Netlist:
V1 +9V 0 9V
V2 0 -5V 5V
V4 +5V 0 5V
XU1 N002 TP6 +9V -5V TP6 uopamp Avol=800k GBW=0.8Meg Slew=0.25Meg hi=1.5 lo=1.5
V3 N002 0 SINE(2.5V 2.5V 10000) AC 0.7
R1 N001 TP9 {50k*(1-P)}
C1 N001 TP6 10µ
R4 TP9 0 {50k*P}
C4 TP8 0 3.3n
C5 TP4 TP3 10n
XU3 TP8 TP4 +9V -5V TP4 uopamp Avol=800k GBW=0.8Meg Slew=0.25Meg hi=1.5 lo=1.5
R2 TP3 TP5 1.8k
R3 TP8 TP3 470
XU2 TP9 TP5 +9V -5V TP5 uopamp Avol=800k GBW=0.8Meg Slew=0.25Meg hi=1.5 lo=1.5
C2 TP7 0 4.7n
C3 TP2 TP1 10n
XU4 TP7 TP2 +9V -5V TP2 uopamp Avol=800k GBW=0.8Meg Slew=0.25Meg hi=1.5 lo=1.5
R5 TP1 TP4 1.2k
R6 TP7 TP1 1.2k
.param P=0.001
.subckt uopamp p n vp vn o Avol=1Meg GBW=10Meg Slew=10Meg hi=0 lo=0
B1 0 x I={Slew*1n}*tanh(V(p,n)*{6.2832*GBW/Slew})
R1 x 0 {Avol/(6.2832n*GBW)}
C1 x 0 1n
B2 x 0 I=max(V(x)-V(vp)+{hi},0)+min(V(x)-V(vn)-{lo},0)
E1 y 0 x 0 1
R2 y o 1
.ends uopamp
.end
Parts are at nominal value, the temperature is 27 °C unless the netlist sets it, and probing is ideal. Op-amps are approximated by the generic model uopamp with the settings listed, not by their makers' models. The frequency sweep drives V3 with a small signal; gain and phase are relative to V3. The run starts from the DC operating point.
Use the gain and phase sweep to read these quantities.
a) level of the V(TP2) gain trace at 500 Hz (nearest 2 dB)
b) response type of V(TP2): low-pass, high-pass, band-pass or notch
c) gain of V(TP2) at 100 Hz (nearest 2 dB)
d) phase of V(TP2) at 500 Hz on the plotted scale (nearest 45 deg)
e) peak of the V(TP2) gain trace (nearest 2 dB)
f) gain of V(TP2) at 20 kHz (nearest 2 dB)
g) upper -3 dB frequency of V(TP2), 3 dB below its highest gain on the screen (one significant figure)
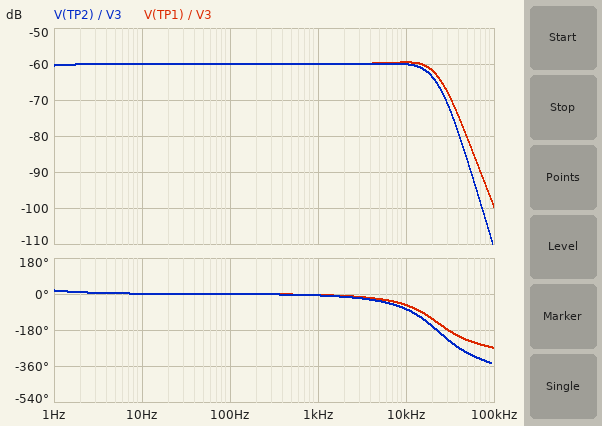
-60 dB
low-pass
-60 dB
0 deg
-60 dB
-64 dB
20 kHz
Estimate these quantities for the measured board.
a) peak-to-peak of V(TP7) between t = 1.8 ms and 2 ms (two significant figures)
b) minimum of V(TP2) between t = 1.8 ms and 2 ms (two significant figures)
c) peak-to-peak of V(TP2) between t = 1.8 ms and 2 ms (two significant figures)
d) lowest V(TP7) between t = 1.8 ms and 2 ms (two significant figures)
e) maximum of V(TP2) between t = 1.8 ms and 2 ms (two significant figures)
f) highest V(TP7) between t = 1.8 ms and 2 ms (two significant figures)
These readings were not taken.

5.0 mV
-2.5 mV
5.0 mV
-2.5 mV
2.5 mV
2.5 mV
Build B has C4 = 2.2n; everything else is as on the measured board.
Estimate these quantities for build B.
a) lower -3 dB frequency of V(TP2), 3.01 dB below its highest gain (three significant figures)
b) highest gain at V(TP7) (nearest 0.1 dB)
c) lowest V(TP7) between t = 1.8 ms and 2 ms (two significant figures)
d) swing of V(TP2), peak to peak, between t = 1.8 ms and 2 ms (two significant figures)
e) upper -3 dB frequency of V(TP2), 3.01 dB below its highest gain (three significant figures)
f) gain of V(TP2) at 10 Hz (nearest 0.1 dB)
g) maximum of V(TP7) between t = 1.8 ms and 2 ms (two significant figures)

335 mHz
-59.8 dB
-2.6 mV
5.1 mV
21.3 kHz
-60.0 dB
2.6 mV
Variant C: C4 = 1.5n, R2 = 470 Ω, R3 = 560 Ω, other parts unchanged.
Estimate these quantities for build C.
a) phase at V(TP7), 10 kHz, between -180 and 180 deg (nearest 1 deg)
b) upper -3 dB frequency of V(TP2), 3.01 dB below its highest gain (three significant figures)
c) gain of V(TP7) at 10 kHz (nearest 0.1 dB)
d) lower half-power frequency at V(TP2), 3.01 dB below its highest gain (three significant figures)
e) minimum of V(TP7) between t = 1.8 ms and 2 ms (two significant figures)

-52 deg
20.8 kHz
-60.0 dB
325 mHz
-2.5 mV
